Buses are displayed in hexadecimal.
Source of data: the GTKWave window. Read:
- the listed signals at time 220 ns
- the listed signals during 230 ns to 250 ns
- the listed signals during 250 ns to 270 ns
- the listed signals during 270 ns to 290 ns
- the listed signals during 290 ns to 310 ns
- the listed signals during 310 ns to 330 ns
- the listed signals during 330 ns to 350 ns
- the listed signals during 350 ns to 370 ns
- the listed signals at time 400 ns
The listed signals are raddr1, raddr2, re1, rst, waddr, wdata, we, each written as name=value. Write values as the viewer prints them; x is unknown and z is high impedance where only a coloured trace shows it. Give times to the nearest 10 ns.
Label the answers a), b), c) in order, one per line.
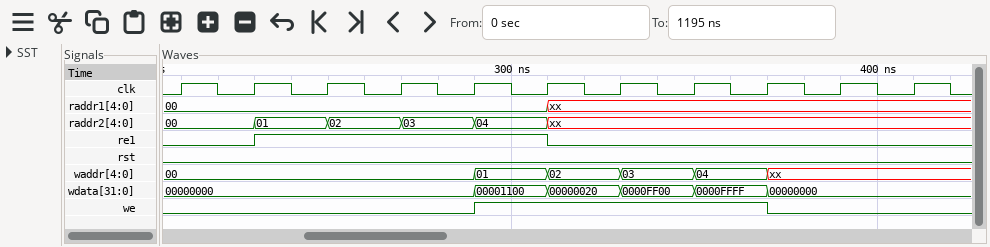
a) raddr1=00, raddr2=00, re1=0, rst=0, waddr=00, wdata=00000000, we=0
b) raddr1=00, raddr2=01, re1=1, rst=0, waddr=00, wdata=00000000, we=0
c) raddr1=00, raddr2=02, re1=1, rst=0, waddr=00, wdata=00000000, we=0
d) raddr1=00, raddr2=03, re1=1, rst=0, waddr=00, wdata=00000000, we=0
e) raddr1=00, raddr2=04, re1=1, rst=0, waddr=01, wdata=00001100, we=1
f) raddr1=xx, raddr2=xx, re1=0, rst=0, waddr=02, wdata=00000020, we=1
g) raddr1=xx, raddr2=xx, re1=0, rst=0, waddr=03, wdata=0000FF00, we=1
h) raddr1=xx, raddr2=xx, re1=0, rst=0, waddr=04, wdata=0000FFFF, we=1
i) raddr1=xx, raddr2=xx, re1=0, rst=0, waddr=xx, wdata=00000000, we=0
